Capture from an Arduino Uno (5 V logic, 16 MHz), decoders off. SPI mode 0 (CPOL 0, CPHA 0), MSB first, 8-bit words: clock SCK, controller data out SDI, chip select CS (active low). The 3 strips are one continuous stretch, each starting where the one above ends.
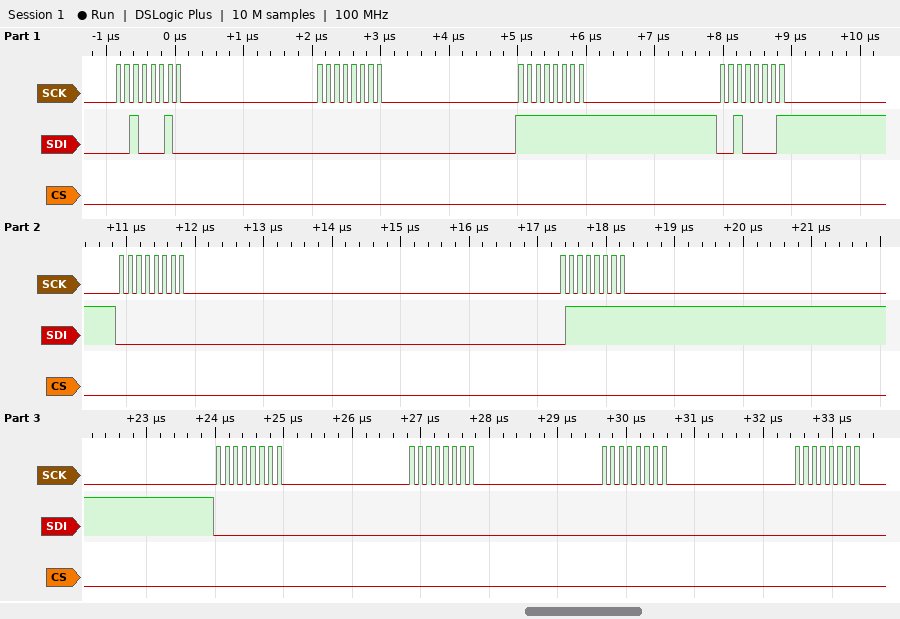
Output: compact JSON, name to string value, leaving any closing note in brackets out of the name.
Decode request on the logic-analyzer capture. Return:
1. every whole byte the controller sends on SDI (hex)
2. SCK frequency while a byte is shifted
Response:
{"every whole byte the controller sends on SDI": "0x22 0x00 0xFF 0x21 0x00 0x7F 0x00 0x00 0x00 0x00", "SCK frequency while a byte is shifted": "8 MHz"}
